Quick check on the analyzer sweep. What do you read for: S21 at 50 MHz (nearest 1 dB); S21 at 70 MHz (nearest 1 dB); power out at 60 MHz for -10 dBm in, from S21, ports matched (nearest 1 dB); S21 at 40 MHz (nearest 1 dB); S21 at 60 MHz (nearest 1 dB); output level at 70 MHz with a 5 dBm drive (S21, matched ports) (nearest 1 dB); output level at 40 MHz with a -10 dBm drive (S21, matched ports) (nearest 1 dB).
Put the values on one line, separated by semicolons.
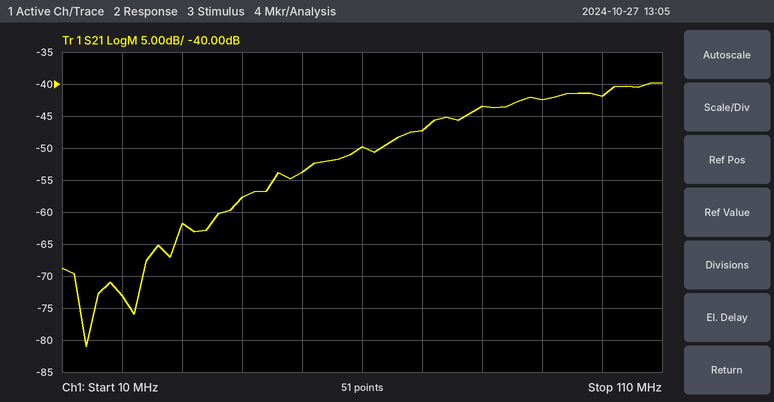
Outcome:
-54 dB; -47 dB; -60 dBm; -58 dB; -50 dB; -42 dBm; -68 dBm
